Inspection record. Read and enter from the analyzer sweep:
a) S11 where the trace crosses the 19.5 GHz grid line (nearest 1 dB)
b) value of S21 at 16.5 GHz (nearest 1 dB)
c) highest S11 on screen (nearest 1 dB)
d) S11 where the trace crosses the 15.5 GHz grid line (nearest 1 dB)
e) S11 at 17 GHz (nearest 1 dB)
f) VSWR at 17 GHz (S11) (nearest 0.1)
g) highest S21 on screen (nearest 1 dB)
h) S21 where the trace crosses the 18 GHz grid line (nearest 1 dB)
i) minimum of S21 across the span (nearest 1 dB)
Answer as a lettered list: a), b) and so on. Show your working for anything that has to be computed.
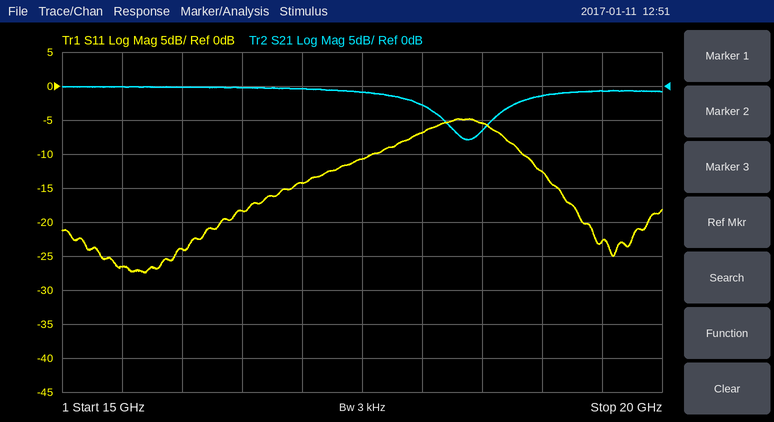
a) -23 dB
b) 0 dB
c) -5 dB
d) -27 dB
e) -14 dB
f) |Γ| = 10^(-14/20) = 0.1995; VSWR = (1 + 0.1995)/(1 − 0.1995) ≈ 1.5
g) 0 dB
h) -3 dB
i) -8 dB
